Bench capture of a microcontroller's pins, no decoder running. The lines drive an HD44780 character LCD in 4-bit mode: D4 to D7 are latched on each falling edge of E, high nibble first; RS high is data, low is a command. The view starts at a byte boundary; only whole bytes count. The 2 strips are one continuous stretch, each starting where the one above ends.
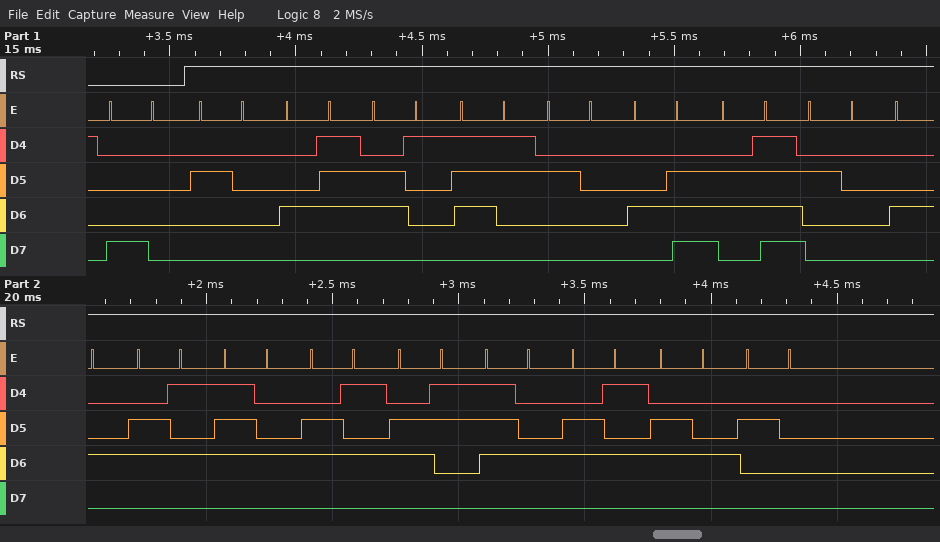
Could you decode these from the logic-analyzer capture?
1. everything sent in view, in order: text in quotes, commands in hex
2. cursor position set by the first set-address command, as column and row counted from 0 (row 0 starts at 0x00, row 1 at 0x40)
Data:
0x80 " Gas No Detected "
column 0, row 0
